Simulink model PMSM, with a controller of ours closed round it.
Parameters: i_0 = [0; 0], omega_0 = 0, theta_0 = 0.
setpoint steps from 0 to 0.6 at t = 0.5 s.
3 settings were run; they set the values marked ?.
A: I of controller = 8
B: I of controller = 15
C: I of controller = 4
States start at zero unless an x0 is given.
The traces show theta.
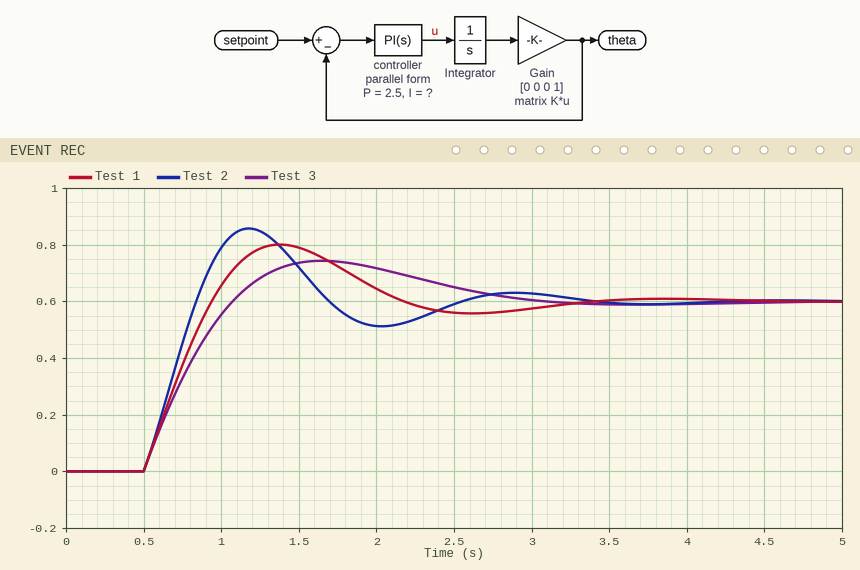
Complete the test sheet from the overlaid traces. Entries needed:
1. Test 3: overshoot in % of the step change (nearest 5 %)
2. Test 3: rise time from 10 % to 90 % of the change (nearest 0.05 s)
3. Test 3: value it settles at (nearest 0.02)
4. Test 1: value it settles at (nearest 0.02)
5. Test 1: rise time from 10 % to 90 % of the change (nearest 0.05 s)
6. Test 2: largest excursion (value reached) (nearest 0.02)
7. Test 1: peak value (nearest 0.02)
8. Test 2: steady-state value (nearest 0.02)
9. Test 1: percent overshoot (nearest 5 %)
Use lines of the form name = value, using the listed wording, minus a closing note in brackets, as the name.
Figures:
Test 3: overshoot in % of the step change = 25 %
Test 3: rise time from 10 % to 90 % of the change = 0.45 s
Test 3: value it settles at = 0.60
Test 1: value it settles at = 0.60
Test 1: rise time from 10 % to 90 % of the change = 0.35 s
Test 2: largest excursion (value reached) = 0.86
Test 1: peak value = 0.80
Test 2: steady-state value = 0.60
Test 1: percent overshoot = 35 %
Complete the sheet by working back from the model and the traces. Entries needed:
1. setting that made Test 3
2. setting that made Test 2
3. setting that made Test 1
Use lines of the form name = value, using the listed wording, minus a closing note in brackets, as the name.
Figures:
setting that made Test 3 = C
setting that made Test 2 = B
setting that made Test 1 = A
